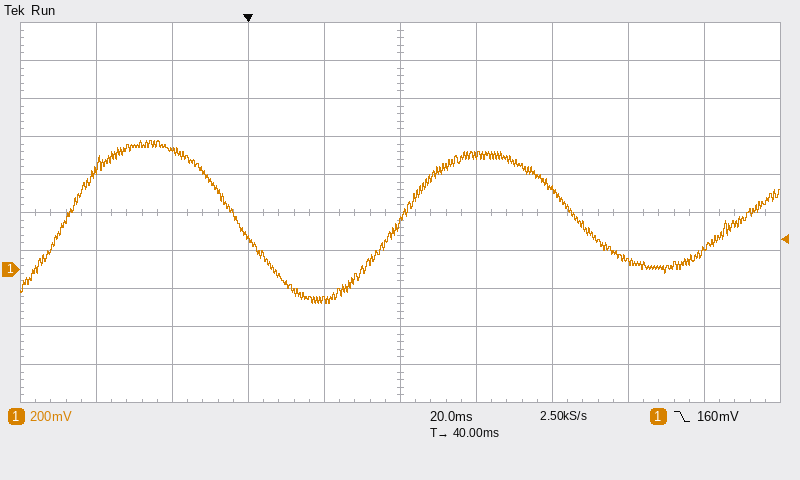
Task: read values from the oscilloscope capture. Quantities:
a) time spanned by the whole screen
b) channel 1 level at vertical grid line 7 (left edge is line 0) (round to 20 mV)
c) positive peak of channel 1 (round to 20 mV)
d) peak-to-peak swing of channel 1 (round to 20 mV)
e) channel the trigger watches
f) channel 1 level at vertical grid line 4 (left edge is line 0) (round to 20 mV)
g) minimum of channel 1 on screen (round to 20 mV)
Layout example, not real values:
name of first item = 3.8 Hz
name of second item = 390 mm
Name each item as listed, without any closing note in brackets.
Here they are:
time spanned by the whole screen = 200 ms
channel 1 level at vertical grid line 7 (left edge is line 0) = 420 mV
positive peak of channel 1 = 680 mV
peak-to-peak swing of channel 1 = 860 mV
channel the trigger watches = channel 1
channel 1 level at vertical grid line 4 (left edge is line 0) = -160 mV
minimum of channel 1 on screen = -180 mV
